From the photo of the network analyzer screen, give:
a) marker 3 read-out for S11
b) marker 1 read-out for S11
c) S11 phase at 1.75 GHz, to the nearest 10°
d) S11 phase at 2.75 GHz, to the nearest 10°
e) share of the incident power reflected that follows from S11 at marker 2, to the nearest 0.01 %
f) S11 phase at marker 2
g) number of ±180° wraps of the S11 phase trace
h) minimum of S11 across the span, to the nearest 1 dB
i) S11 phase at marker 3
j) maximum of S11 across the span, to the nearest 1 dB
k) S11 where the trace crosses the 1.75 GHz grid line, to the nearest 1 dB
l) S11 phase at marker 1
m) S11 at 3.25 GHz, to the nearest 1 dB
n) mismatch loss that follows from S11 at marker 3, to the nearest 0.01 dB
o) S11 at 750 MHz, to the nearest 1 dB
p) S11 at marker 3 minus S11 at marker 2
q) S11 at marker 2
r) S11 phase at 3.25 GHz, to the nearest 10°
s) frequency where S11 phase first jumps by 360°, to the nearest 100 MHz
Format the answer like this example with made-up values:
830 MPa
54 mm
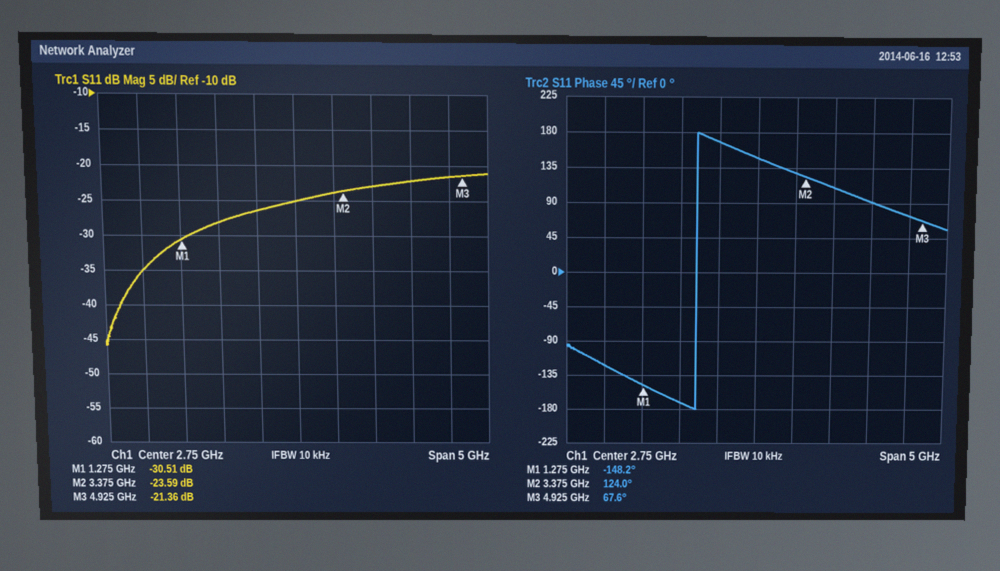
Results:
-21.36 dB
-30.51 dB
-170°
150°
0.44 %
124.0°
1
-46 dB
67.6°
-21 dB
-28 dB
-148.2°
-24 dB
0.03 dB
-35 dB
2.23 dB
-23.59 dB
130°
2.0 GHz
